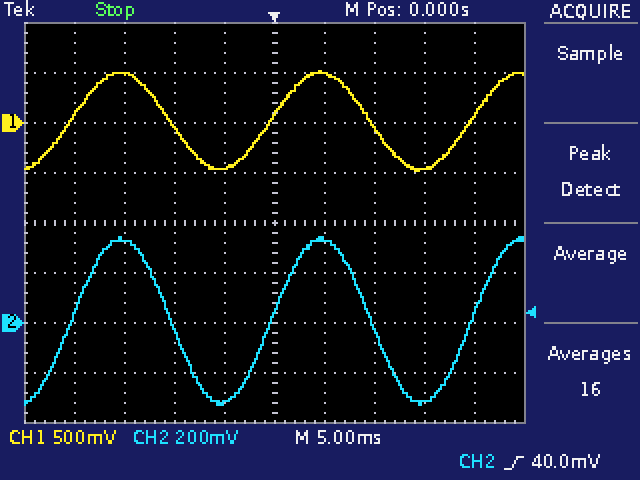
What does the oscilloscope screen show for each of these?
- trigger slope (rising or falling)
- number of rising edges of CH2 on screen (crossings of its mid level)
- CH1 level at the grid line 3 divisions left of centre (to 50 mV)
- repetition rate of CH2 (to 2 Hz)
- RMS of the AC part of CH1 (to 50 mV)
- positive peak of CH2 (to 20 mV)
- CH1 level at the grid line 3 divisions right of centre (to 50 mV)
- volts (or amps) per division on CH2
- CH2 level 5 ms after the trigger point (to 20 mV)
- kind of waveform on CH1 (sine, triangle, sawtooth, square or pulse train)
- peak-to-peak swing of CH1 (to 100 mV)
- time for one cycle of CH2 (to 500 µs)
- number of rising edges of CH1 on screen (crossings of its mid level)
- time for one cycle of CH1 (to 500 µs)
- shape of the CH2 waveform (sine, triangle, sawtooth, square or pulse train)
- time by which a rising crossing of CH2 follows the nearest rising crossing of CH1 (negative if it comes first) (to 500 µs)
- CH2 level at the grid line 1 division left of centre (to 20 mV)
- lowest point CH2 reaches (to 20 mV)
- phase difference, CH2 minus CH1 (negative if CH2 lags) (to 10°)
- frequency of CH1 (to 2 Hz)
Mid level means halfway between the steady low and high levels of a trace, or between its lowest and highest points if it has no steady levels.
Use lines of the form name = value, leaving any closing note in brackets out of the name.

trigger slope = rising
number of rising edges of CH2 on screen = 3
CH1 level at the grid line 3 divisions left of centre = 500 mV
repetition rate of CH2 = 50 Hz
RMS of the AC part of CH1 = 350 mV
positive peak of CH2 = 340 mV
CH1 level at the grid line 3 divisions right of centre = -450 mV
volts (or amps) per division on CH2 = 200 mV
CH2 level 5 ms after the trigger point = 340 mV
kind of waveform on CH1 = sine
peak-to-peak swing of CH1 = 1.00 V
time for one cycle of CH2 = 20.0 ms
number of rising edges of CH1 on screen = 3
time for one cycle of CH1 = 20.0 ms
shape of the CH2 waveform = sine
time by which a rising crossing of CH2 follows the nearest rising crossing of CH1 (negative if it comes first) = 0.0 ms
CH2 level at the grid line 1 division left of centre = -320 mV
lowest point CH2 reaches = -320 mV
phase difference, CH2 minus CH1 (negative if CH2 lags) = 0°
frequency of CH1 = 50 Hz
